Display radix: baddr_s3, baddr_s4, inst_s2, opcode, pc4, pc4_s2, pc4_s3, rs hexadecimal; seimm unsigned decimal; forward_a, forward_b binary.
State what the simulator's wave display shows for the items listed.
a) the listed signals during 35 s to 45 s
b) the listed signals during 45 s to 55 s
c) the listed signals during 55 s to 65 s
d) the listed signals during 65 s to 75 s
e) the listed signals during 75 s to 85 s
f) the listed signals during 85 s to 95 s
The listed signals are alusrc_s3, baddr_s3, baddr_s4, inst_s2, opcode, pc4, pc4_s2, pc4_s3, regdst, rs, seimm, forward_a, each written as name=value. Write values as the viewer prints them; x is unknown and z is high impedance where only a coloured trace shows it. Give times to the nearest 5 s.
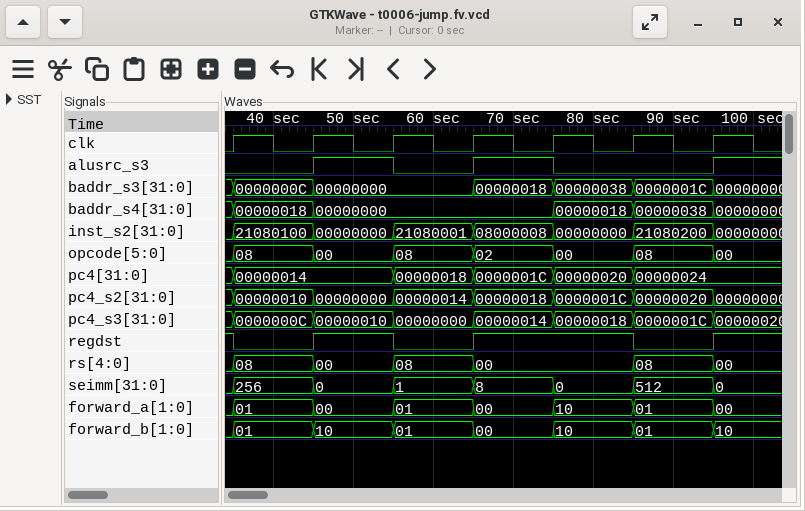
alusrc_s3=0, baddr_s3=0000000C, baddr_s4=00000018, inst_s2=21080100, opcode=08, pc4=00000014, pc4_s2=00000010, pc4_s3=0000000C, regdst=0, rs=08, seimm=256, forward_a=01
alusrc_s3=1, baddr_s3=00000000, baddr_s4=00000000, inst_s2=00000000, opcode=00, pc4=00000014, pc4_s2=00000000, pc4_s3=00000010, regdst=1, rs=00, seimm=0, forward_a=00
alusrc_s3=0, baddr_s3=00000000, baddr_s4=00000000, inst_s2=21080001, opcode=08, pc4=00000018, pc4_s2=00000014, pc4_s3=00000000, regdst=0, rs=08, seimm=1, forward_a=01
alusrc_s3=1, baddr_s3=00000018, baddr_s4=00000000, inst_s2=08000008, opcode=02, pc4=0000001C, pc4_s2=00000018, pc4_s3=00000014, regdst=1, rs=00, seimm=8, forward_a=00
alusrc_s3=0, baddr_s3=00000038, baddr_s4=00000018, inst_s2=00000000, opcode=00, pc4=00000020, pc4_s2=0000001C, pc4_s3=00000018, regdst=1, rs=00, seimm=0, forward_a=10
alusrc_s3=0, baddr_s3=0000001C, baddr_s4=00000038, inst_s2=21080200, opcode=08, pc4=00000024, pc4_s2=00000020, pc4_s3=0000001C, regdst=0, rs=08, seimm=512, forward_a=01
